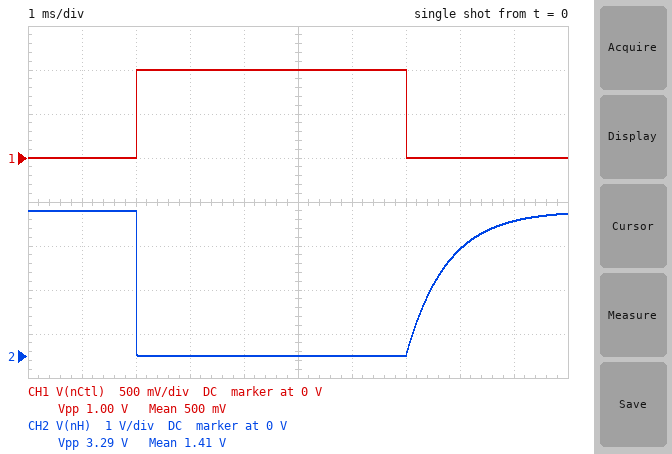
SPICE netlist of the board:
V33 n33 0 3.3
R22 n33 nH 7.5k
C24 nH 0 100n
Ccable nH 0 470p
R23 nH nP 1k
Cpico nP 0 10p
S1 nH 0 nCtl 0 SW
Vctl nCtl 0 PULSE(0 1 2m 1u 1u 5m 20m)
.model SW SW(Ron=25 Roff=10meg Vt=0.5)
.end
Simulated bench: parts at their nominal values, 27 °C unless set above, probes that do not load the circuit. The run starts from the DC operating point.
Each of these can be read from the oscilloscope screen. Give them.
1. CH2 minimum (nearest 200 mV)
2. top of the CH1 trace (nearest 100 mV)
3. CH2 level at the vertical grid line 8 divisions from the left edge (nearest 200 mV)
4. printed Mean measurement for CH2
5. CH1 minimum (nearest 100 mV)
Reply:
0 V
1.0 V
2.4 V
1.41 V
0 V
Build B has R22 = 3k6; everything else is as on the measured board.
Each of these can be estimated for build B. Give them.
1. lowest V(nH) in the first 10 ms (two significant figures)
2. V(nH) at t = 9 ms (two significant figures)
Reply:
23 mV
3.3 V
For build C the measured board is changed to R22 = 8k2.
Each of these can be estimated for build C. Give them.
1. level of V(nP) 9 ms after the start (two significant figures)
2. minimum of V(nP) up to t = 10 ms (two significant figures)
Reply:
3.0 V
10 mV
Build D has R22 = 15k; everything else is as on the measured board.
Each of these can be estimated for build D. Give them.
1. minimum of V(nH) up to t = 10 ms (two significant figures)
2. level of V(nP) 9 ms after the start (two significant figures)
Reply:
5.5 mV
2.4 V
